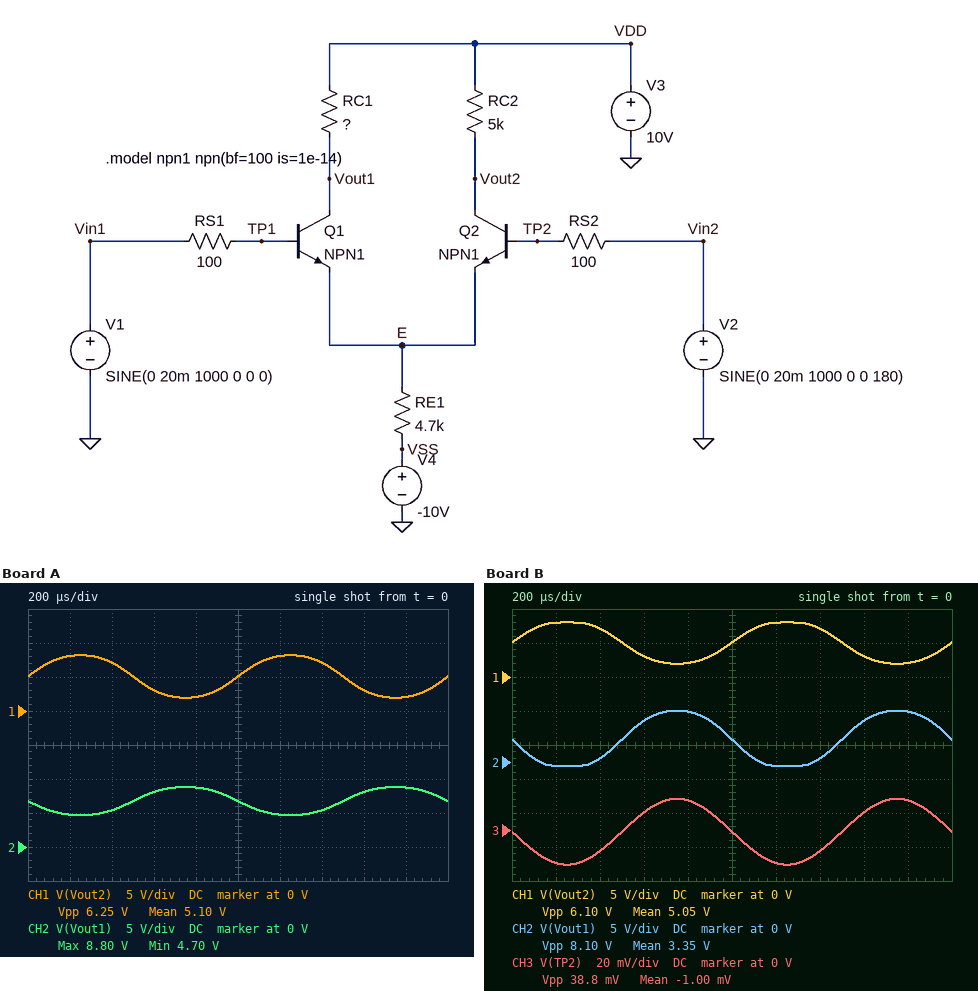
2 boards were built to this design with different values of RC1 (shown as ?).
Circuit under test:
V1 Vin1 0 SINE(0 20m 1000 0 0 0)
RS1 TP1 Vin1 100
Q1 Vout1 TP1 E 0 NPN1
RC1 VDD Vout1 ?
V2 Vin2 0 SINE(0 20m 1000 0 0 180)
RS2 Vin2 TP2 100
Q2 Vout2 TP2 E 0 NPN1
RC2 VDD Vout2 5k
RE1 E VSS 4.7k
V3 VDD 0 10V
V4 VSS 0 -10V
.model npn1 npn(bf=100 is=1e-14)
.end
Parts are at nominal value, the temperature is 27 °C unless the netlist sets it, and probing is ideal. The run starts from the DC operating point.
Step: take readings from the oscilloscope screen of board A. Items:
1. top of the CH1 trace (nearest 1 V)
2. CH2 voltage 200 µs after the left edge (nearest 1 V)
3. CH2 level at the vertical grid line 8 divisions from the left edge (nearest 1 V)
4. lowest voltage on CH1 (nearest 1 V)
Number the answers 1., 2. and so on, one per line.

1. 8 V
2. 5 V
3. 8 V
4. 2 V
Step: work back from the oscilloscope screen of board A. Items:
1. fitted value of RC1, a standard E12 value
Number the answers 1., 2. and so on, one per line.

1. 3.3 kΩ
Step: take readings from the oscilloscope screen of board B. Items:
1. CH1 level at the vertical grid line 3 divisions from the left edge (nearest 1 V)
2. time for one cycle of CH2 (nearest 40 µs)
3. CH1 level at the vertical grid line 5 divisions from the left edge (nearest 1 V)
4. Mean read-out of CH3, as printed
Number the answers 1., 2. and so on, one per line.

1. 3 V
2. 1.00 ms
3. 5 V
4. -1.00 mV
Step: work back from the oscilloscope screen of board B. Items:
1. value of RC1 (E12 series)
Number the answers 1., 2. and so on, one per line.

1. 6.8 kΩ
